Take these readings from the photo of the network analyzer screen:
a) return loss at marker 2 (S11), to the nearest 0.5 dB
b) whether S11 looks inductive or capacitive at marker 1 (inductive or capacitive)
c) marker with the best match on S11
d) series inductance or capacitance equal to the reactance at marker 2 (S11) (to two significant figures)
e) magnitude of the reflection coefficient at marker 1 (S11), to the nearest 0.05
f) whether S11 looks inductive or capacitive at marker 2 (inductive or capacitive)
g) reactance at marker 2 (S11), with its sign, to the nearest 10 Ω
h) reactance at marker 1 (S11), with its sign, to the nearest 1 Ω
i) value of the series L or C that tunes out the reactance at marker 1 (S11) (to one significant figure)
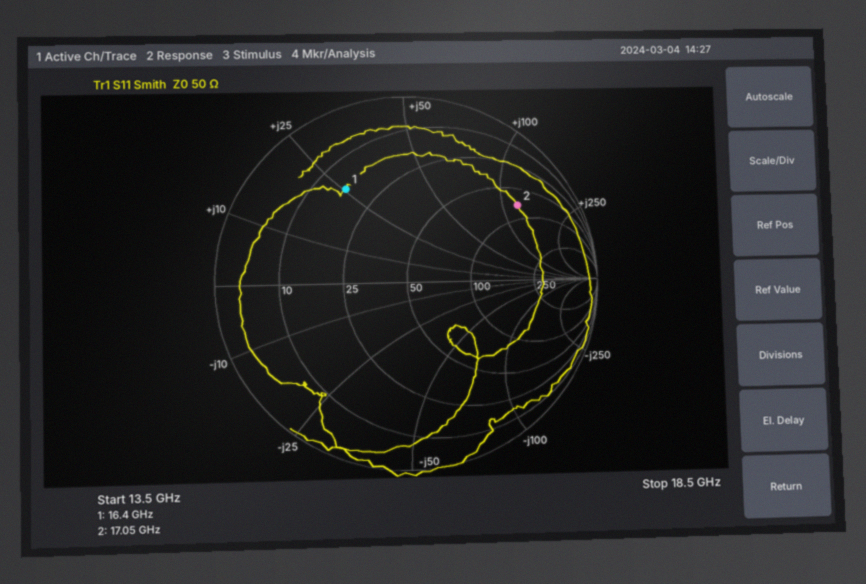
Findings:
3.0 dB
inductive
marker 1
1.1 nH
0.60
inductive
+120 Ω
+26 Ω
400 fF
